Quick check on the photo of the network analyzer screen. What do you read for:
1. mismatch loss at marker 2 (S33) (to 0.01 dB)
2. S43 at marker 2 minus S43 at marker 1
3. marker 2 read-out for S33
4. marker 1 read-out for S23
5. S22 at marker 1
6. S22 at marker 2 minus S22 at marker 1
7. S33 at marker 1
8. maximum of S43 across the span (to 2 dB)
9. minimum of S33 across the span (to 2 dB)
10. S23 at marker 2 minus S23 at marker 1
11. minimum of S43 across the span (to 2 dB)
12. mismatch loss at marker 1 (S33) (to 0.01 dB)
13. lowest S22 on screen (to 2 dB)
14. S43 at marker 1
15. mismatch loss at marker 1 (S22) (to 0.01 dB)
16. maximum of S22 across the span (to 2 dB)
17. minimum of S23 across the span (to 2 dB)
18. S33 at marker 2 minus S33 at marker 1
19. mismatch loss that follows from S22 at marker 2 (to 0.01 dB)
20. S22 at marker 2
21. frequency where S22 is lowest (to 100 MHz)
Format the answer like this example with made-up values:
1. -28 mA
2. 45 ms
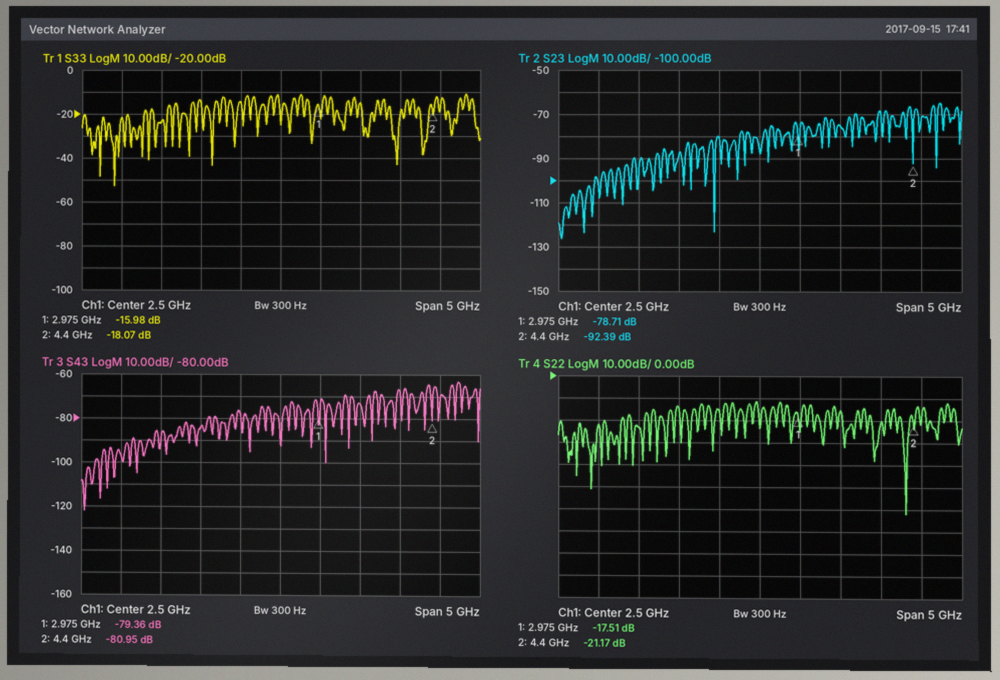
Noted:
1. 0.07 dB
2. -1.59 dB
3. -18.07 dB
4. -78.71 dB
5. -17.51 dB
6. -3.66 dB
7. -15.98 dB
8. -64 dB
9. -52 dB
10. -13.68 dB
11. -122 dB
12. 0.11 dB
13. -62 dB
14. -79.36 dB
15. 0.08 dB
16. -12 dB
17. -126 dB
18. -2.09 dB
19. 0.03 dB
20. -21.17 dB
21. 4.3 GHz
